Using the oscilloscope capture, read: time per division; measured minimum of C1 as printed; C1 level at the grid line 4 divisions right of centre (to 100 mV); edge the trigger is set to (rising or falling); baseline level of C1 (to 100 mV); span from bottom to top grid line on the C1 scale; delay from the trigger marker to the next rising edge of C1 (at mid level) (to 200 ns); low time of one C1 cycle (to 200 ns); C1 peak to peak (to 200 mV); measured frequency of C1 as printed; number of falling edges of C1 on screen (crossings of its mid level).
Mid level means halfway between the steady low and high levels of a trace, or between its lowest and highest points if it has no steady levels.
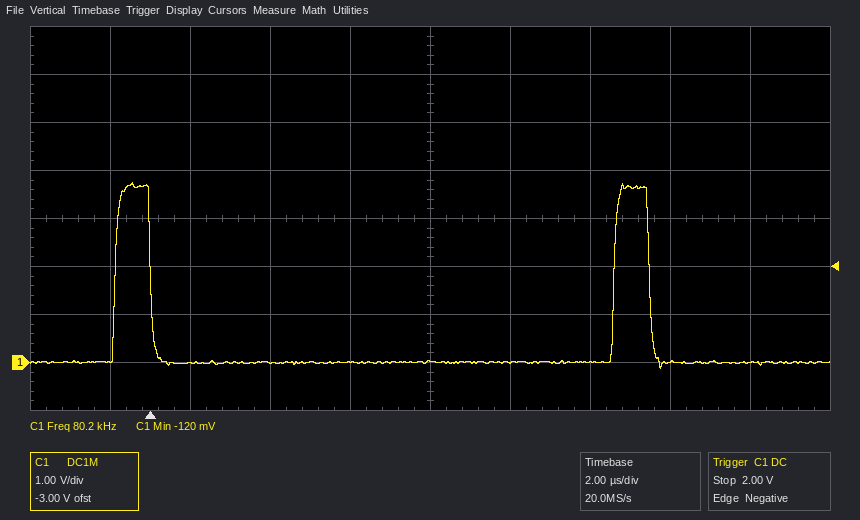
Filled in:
2 µs
-120 mV
0.0 V
falling
0.0 V
8 V
11.6 µs
11.6 µs
3.8 V
80.2 kHz
2
